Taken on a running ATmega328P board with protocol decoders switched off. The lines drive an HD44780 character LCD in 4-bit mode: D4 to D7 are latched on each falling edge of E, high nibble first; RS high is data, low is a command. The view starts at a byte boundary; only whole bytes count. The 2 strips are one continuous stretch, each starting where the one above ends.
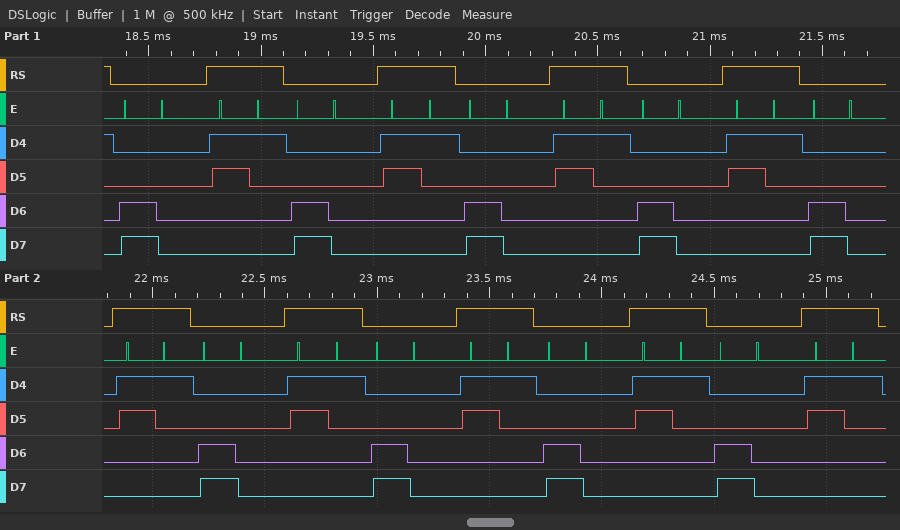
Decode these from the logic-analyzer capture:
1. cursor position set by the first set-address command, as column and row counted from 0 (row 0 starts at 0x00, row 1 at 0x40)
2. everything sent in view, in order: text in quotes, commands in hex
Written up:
column 0, row 1
0xC0 "1" 0xC0 "1" 0xC0 "1" 0xC0 "1" 0xC0 "1" 0xC0 "1" 0xC0 "1" 0xC0 "1" 0xC0 "1"
